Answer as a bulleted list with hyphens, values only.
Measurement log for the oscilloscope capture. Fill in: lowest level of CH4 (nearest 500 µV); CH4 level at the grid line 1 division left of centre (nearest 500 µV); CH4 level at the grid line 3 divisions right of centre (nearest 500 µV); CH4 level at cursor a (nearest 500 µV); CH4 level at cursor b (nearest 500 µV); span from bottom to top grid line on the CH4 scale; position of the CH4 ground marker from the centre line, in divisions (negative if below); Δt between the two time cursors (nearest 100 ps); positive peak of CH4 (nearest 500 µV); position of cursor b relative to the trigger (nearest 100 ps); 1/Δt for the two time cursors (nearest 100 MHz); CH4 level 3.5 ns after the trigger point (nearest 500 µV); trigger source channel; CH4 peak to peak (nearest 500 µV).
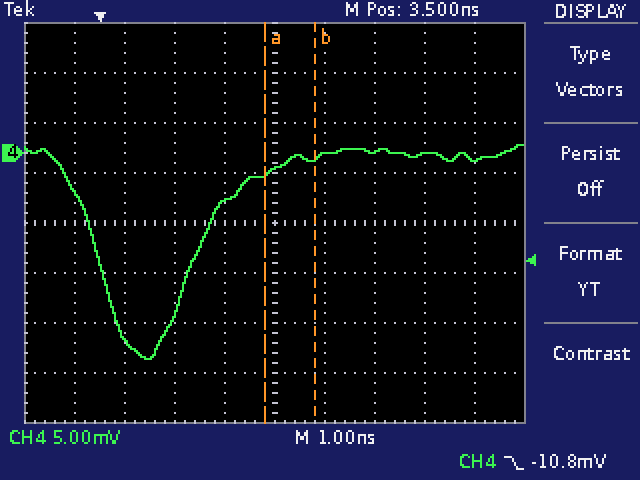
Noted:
- -20.5 mV
- -5.0 mV
- 0.0 mV
- -2.0 mV
- -500 µV
- 40 mV
- +1.4 div
- 1.0 ns
- 1.0 mV
- +4.3 ns
- 1.0 GHz
- -1.5 mV
- CH4
- 21.5 mV
